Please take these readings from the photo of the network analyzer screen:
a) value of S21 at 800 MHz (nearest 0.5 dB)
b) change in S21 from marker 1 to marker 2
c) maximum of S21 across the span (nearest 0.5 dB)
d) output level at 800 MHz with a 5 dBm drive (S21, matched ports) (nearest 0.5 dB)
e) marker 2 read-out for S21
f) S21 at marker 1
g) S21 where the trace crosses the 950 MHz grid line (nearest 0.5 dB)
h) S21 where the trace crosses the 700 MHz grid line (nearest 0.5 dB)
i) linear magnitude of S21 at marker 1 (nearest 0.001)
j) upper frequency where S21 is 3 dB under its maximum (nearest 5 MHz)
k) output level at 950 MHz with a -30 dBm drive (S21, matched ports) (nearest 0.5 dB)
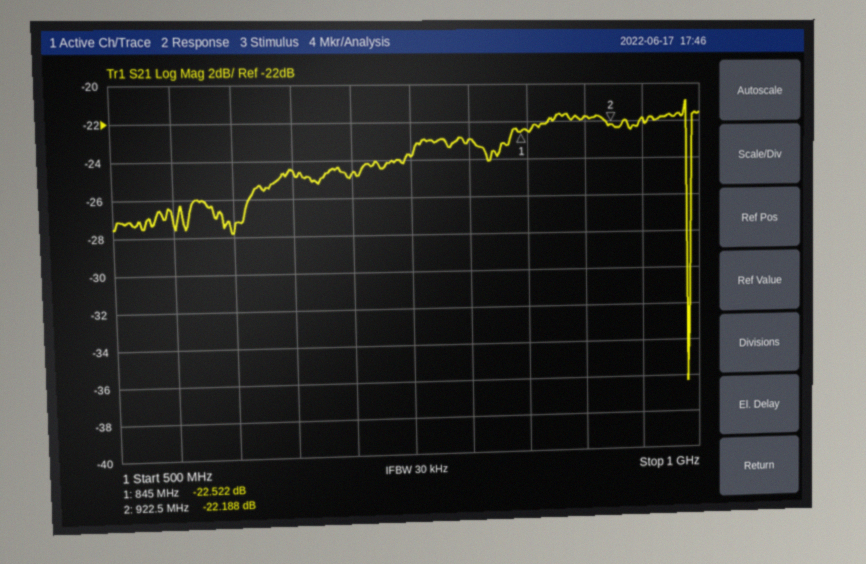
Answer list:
-23.0 dB
0.334 dB
-21.0 dB
-18.0 dBm
-22.188 dB
-22.522 dB
-22.0 dB
-24.5 dB
0.075
990 MHz
-52.0 dBm
